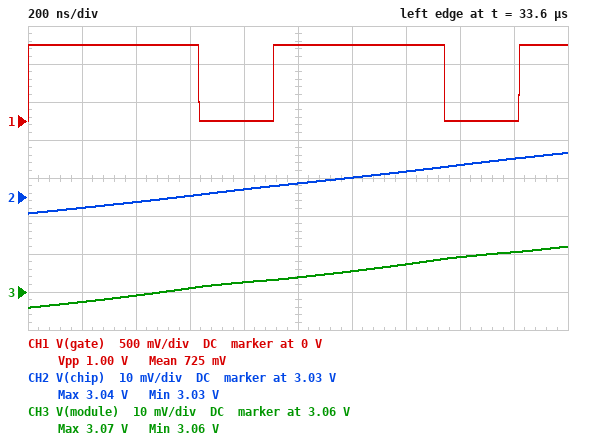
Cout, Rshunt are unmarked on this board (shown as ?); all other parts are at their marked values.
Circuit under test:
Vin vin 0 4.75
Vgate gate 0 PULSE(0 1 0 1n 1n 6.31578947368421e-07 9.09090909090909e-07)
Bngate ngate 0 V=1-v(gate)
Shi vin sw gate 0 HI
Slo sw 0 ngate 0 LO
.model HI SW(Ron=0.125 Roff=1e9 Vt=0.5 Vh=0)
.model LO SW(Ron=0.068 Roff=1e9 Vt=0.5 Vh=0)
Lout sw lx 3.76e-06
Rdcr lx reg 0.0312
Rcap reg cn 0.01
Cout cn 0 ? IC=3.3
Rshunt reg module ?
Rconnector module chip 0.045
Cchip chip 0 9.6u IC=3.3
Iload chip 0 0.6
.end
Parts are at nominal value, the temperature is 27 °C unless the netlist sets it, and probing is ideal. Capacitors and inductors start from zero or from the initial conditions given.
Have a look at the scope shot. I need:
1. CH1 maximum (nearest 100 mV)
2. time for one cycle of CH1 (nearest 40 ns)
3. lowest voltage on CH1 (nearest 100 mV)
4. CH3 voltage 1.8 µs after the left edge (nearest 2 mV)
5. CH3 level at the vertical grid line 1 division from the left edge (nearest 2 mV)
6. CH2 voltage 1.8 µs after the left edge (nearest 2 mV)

1.0 V
920 ns
0 V
3.070 V
3.058 V
3.040 V
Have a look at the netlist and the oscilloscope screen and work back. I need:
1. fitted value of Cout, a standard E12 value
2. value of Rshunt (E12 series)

18 µF
0.18 Ω
